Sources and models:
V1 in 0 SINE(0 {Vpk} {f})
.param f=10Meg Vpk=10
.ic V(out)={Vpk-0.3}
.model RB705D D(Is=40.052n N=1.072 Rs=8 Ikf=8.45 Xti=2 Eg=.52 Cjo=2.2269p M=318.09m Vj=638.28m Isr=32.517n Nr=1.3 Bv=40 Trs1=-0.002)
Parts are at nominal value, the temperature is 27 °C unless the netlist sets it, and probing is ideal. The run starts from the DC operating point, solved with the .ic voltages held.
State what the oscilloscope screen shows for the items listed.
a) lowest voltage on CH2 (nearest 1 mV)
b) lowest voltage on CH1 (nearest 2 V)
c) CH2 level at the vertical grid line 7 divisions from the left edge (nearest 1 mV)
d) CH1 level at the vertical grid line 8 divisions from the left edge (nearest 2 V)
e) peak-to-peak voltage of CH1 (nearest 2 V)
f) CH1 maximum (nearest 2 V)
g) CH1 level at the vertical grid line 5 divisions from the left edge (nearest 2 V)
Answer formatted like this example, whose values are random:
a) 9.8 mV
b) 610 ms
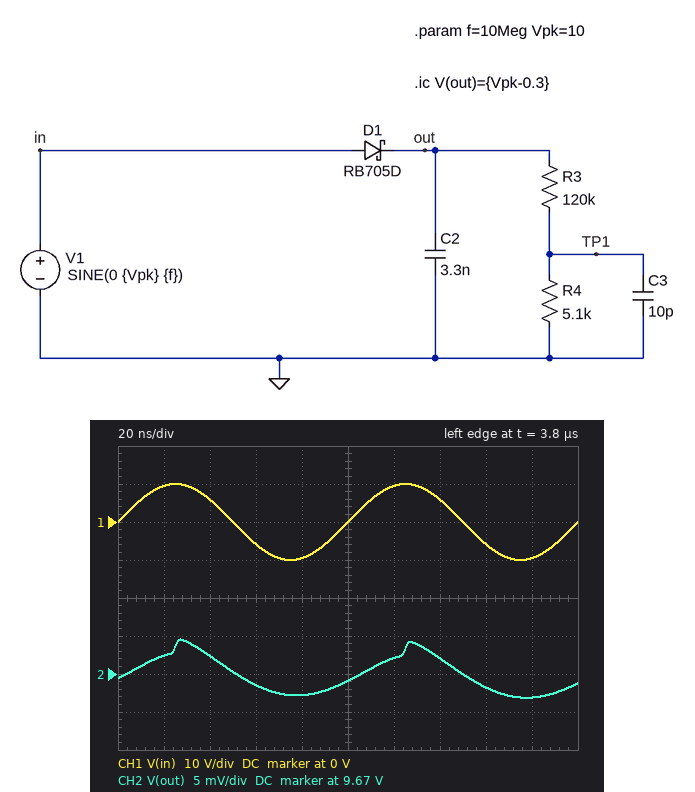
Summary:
a) 9.667 V
b) -10 V
c) 9.672 V
d) -6 V
e) 20 V
f) 10 V
g) 0 V
